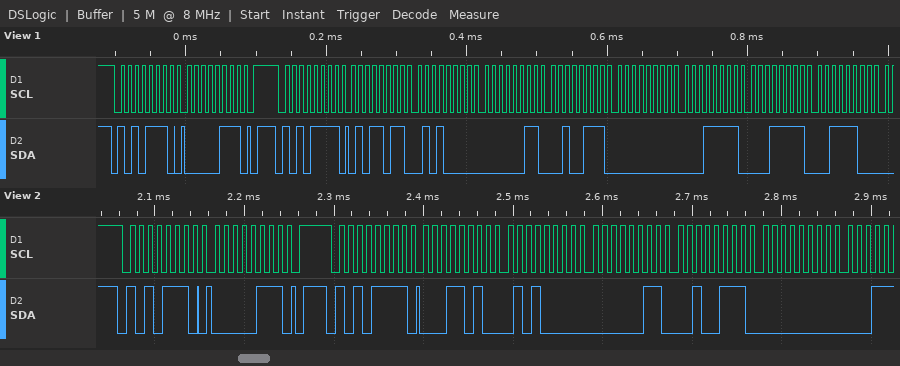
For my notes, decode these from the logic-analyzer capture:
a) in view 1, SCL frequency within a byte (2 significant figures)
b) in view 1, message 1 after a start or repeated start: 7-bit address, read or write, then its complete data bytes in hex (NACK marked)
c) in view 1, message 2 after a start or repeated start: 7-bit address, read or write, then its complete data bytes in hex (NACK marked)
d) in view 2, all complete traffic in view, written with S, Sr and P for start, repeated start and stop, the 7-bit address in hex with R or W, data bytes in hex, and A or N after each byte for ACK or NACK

100 kHz
0x57 write: 07
0x57 read: 5B 50 03 27 00 1F 1F 3C
S 57W A 07 A P S 57R A 1A A 50 A 03 A 27 A 00 A
